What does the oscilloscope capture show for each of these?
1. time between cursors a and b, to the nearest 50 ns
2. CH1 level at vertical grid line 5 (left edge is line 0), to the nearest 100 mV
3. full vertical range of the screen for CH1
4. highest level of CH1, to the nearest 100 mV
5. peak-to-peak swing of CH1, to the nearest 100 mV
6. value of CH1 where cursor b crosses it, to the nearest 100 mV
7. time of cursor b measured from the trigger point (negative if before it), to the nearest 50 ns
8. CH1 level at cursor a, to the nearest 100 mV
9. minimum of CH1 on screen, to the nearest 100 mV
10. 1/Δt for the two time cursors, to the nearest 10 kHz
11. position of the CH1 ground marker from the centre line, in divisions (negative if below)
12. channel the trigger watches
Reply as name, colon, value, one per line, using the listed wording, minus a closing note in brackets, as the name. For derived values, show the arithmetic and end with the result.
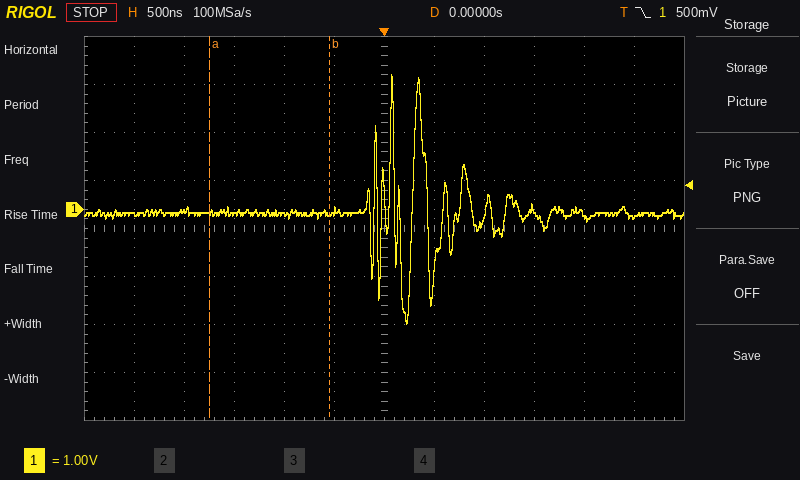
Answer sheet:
time between cursors a and b, to the nearest 50 ns: 1.20 µs
CH1 level at vertical grid line 5 (left edge is line 0), to the nearest 100 mV: 0.0 V
full vertical range of the screen for CH1: 8 V
highest level of CH1, to the nearest 100 mV: 2.8 V
peak-to-peak swing of CH1, to the nearest 100 mV: 2.8 V − (-2.4 V) = 5.2 V
value of CH1 where cursor b crosses it, to the nearest 100 mV: -100 mV
time of cursor b measured from the trigger point (negative if before it), to the nearest 50 ns: -550 ns
CH1 level at cursor a, to the nearest 100 mV: -100 mV
minimum of CH1 on screen, to the nearest 100 mV: -2.4 V
1/Δt for the two time cursors, to the nearest 10 kHz: 1 / 1.20 µs ≈ 830 kHz
position of the CH1 ground marker from the centre line, in divisions: +0.4 div
channel the trigger watches: CH1
